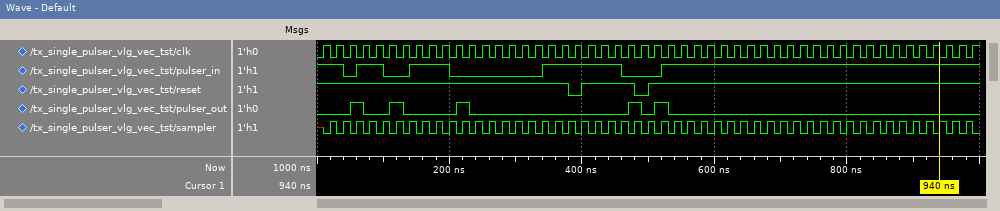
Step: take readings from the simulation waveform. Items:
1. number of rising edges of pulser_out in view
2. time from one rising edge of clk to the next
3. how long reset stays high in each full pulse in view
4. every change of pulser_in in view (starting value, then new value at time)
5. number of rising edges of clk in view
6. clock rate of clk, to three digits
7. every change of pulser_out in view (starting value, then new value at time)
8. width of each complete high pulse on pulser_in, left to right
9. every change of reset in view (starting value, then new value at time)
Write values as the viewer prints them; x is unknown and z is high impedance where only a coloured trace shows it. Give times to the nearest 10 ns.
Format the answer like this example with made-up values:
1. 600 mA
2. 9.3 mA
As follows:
1. 5
2. 20 ns
3. 80 ns
4. 1, 0 at 40 ns, 1 at 60 ns, 0 at 100 ns, 1 at 140 ns, 0 at 200 ns, 1 at 340 ns, 0 at 460 ns, 1 at 520 ns
5. 50
6. 50.0 MHz
7. 0, 1 at 50 ns, 0 at 70 ns, 1 at 110 ns, 0 at 130 ns, 1 at 210 ns, 0 at 230 ns, 1 at 470 ns, 0 at 490 ns, 1 at 510 ns, 0 at 530 ns
8. 40 ns, 60 ns, 120 ns
9. 1, 0 at 380 ns, 1 at 400 ns, 0 at 480 ns, 1 at 500 ns
